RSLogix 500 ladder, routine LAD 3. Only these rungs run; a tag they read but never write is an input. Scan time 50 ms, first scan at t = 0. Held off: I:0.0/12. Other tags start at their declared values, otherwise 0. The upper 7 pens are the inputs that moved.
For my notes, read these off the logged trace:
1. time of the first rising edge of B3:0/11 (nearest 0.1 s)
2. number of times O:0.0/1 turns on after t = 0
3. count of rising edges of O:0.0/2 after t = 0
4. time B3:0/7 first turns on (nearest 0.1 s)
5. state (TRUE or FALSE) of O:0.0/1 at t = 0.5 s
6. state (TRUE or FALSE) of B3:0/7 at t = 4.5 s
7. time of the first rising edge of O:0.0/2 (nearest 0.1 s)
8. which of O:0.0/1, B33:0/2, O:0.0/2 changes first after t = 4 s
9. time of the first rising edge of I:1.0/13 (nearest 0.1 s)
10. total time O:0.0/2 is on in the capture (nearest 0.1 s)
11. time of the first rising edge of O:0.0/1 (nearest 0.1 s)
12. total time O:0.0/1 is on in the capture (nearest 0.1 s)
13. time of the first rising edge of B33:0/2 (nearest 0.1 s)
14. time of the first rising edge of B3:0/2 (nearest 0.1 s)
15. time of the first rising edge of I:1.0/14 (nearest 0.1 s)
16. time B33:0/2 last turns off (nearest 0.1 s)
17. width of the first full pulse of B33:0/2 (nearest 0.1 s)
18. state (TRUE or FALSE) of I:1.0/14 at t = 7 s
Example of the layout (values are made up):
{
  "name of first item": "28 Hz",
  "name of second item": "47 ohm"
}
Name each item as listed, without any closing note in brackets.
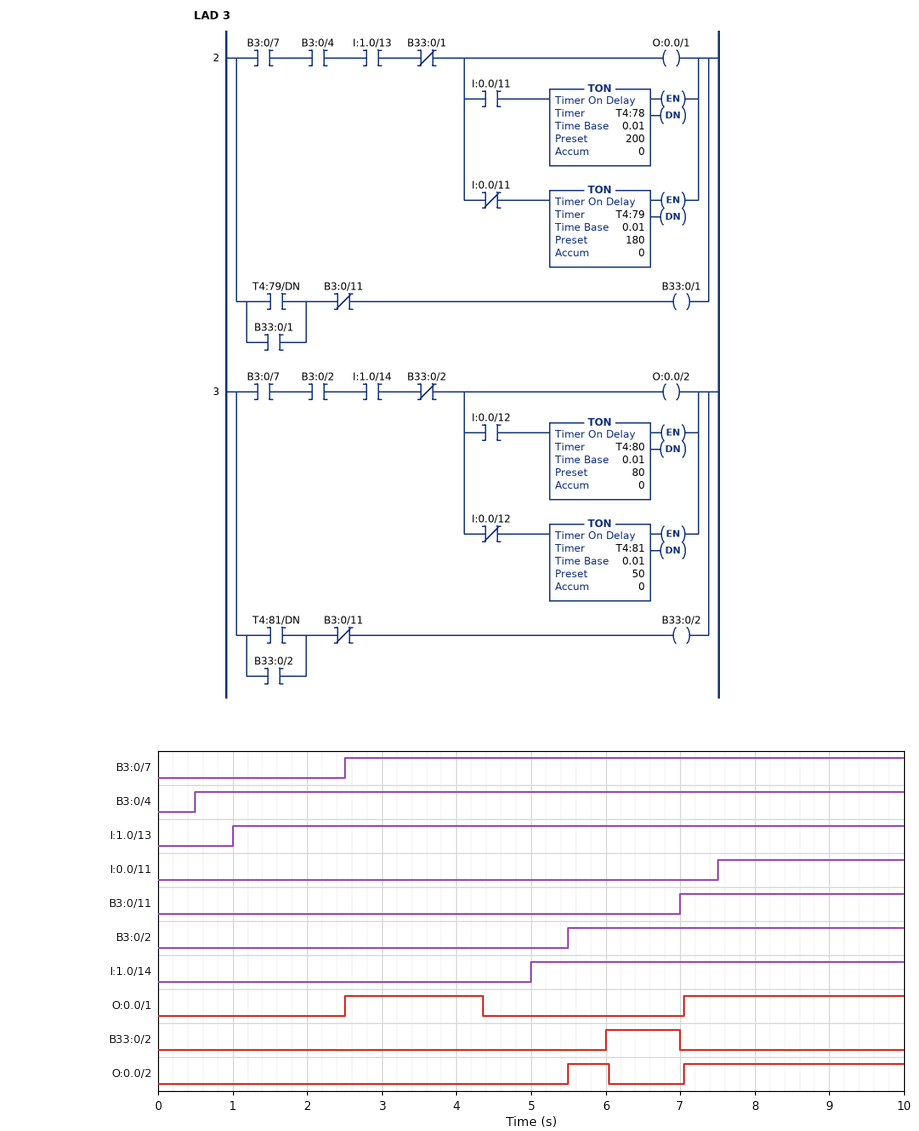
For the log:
{
  "time of the first rising edge of B3:0/11": "7.0 s",
  "number of times O:0.0/1 turns on after t = 0": "2",
  "count of rising edges of O:0.0/2 after t = 0": "2",
  "time B3:0/7 first turns on": "2.5 s",
  "state (TRUE or FALSE) of O:0.0/1 at t = 0.5 s": "FALSE",
  "state (TRUE or FALSE) of B3:0/7 at t = 4.5 s": "TRUE",
  "time of the first rising edge of O:0.0/2": "5.5 s",
  "which of O:0.0/1, B33:0/2, O:0.0/2 changes first after t = 4 s": "O:0.0/1",
  "time of the first rising edge of I:1.0/13": "1.0 s",
  "total time O:0.0/2 is on in the capture": "3.5 s",
  "time of the first rising edge of O:0.0/1": "2.5 s",
  "total time O:0.0/1 is on in the capture": "4.8 s",
  "time of the first rising edge of B33:0/2": "6.0 s",
  "time of the first rising edge of B3:0/2": "5.5 s",
  "time of the first rising edge of I:1.0/14": "5.0 s",
  "time B33:0/2 last turns off": "7.0 s",
  "width of the first full pulse of B33:0/2": "1.0 s",
  "state (TRUE or FALSE) of I:1.0/14 at t = 7 s": "TRUE"
}
